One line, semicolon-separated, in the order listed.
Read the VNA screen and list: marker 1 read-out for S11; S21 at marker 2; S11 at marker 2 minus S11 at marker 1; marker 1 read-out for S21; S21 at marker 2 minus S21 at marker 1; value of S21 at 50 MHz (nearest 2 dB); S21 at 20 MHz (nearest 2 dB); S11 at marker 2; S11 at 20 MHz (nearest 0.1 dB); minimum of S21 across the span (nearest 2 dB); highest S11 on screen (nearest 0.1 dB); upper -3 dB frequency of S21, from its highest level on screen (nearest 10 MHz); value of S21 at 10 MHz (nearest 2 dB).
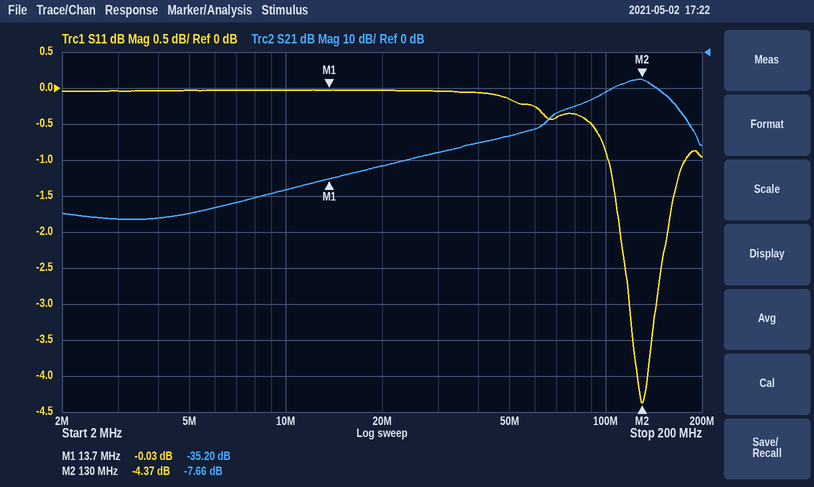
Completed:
-0.03 dB; -7.66 dB; -4.34 dB; -35.20 dB; 27.54 dB; -24 dB; -32 dB; -4.37 dB; 0.0 dB; -46 dB; 0.0 dB; 150 MHz; -38 dB
